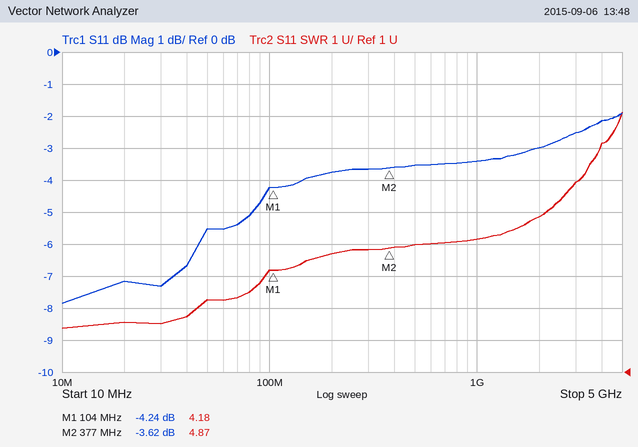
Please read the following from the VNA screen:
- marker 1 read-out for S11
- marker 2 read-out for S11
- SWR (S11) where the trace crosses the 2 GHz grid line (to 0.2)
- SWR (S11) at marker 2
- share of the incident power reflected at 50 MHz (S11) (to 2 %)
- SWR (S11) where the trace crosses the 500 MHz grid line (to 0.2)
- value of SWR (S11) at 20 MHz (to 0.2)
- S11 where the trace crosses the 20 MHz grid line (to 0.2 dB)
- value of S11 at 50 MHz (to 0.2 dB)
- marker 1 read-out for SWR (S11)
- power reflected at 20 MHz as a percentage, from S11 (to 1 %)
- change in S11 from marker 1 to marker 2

-4.24 dB
-3.62 dB
5.8
4.87
28 %
5.0
2.6
-7.2 dB
-5.6 dB
4.18
19 %
0.62 dB
